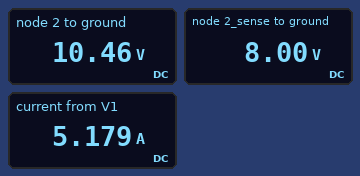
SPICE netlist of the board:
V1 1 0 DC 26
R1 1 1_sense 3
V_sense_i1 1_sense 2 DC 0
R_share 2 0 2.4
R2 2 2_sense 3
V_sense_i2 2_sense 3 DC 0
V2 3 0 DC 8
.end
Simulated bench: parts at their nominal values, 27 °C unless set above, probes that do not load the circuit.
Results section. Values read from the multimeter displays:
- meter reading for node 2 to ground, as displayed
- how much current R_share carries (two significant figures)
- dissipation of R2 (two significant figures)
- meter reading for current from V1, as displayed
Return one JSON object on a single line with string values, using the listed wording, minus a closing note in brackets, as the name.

{"meter reading for node 2 to ground, as displayed": "10.46 V", "how much current R_share carries": "4.4 A", "dissipation of R2": "2.0 W", "meter reading for current from V1, as displayed": "5.179 A"}
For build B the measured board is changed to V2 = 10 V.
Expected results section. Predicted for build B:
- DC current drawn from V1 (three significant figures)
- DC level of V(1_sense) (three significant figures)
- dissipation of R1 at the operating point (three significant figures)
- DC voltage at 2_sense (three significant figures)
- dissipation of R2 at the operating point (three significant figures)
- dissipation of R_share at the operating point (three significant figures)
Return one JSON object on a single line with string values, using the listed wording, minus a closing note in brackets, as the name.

{"DC current drawn from V1": "4.97 A", "DC level of V(1_sense)": "11.1 V", "dissipation of R1 at the operating point": "74.2 W", "DC voltage at 2_sense": "10.0 V", "dissipation of R2 at the operating point": "387 mW", "dissipation of R_share at the operating point": "51.1 W"}
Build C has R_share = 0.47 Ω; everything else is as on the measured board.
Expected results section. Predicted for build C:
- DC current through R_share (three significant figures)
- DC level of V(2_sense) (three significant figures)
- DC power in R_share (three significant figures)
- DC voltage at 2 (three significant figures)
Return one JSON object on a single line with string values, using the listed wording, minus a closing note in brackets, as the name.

{"DC current through R_share": "8.63 A", "DC level of V(2_sense)": "8.00 V", "DC power in R_share": "35.0 W", "DC voltage at 2": "4.06 V"}
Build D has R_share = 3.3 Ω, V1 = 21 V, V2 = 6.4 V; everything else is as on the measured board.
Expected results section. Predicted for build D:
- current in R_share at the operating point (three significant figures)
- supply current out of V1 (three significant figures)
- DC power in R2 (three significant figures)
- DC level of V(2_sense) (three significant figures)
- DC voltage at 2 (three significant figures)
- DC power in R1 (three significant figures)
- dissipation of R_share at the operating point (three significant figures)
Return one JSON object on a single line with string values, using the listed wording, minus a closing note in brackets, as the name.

{"current in R_share at the operating point": "2.85 A", "supply current out of V1": "3.86 A", "DC power in R2": "3.04 W", "DC level of V(2_sense)": "6.40 V", "DC voltage at 2": "9.42 V", "DC power in R1": "44.7 W", "dissipation of R_share at the operating point": "26.9 W"}
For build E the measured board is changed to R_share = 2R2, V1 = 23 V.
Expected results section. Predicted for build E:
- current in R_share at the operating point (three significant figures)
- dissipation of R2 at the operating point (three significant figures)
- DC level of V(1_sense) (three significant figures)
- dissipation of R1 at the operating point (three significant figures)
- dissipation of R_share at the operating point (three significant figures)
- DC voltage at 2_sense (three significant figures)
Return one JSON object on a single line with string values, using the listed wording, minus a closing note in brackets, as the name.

{"current in R_share at the operating point": "4.19 A", "dissipation of R2 at the operating point": "493 mW", "DC level of V(1_sense)": "9.22 V", "dissipation of R1 at the operating point": "63.3 W", "dissipation of R_share at the operating point": "38.6 W", "DC voltage at 2_sense": "8.00 V"}
